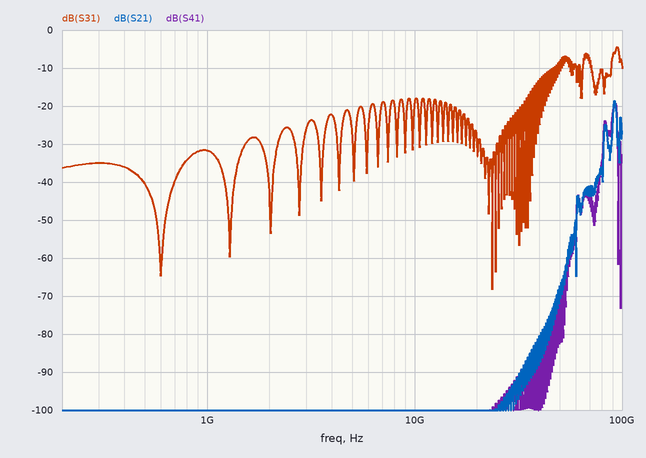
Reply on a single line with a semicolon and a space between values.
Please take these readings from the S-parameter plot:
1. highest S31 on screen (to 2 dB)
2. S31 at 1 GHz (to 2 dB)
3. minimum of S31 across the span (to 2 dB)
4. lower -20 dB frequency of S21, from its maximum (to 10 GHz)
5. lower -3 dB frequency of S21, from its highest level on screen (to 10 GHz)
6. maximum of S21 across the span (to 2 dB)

-4 dB; -32 dB; -68 dB; 80 GHz; 90 GHz; -18 dB
